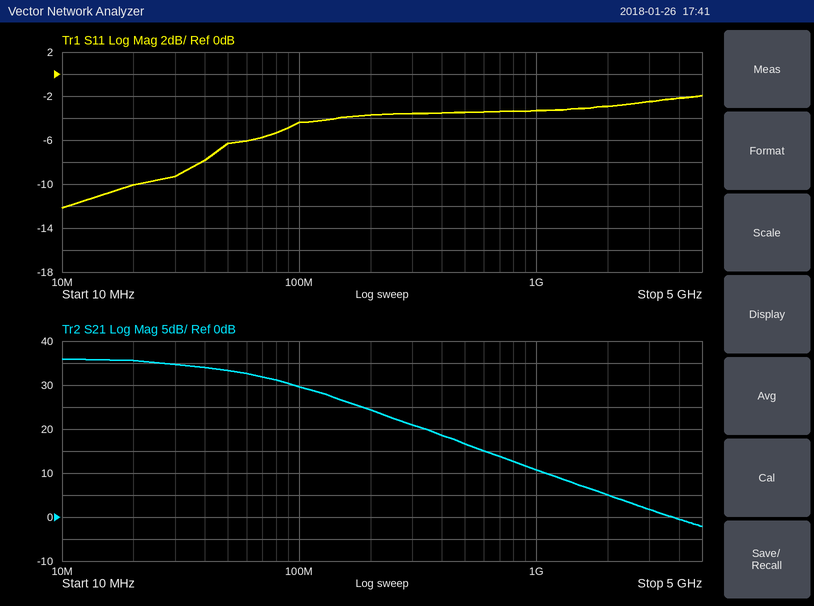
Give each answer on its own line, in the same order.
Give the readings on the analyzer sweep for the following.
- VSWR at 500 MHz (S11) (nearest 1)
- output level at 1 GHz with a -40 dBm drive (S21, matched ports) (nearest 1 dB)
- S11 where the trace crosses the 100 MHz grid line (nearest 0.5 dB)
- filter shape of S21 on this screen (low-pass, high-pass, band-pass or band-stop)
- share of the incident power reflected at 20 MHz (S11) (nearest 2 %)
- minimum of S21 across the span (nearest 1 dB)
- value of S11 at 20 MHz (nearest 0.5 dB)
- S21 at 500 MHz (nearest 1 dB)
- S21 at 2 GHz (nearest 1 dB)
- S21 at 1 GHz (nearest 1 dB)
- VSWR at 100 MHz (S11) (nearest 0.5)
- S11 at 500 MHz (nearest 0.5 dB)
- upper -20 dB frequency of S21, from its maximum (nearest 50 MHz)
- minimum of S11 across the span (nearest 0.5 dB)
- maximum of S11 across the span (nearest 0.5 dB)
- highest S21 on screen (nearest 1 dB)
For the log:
5
-29 dBm
-4.5 dB
low-pass
10 %
-2 dB
-10.0 dB
17 dB
5 dB
11 dB
4.0
-3.5 dB
550 MHz
-12.0 dB
-2.0 dB
36 dB
